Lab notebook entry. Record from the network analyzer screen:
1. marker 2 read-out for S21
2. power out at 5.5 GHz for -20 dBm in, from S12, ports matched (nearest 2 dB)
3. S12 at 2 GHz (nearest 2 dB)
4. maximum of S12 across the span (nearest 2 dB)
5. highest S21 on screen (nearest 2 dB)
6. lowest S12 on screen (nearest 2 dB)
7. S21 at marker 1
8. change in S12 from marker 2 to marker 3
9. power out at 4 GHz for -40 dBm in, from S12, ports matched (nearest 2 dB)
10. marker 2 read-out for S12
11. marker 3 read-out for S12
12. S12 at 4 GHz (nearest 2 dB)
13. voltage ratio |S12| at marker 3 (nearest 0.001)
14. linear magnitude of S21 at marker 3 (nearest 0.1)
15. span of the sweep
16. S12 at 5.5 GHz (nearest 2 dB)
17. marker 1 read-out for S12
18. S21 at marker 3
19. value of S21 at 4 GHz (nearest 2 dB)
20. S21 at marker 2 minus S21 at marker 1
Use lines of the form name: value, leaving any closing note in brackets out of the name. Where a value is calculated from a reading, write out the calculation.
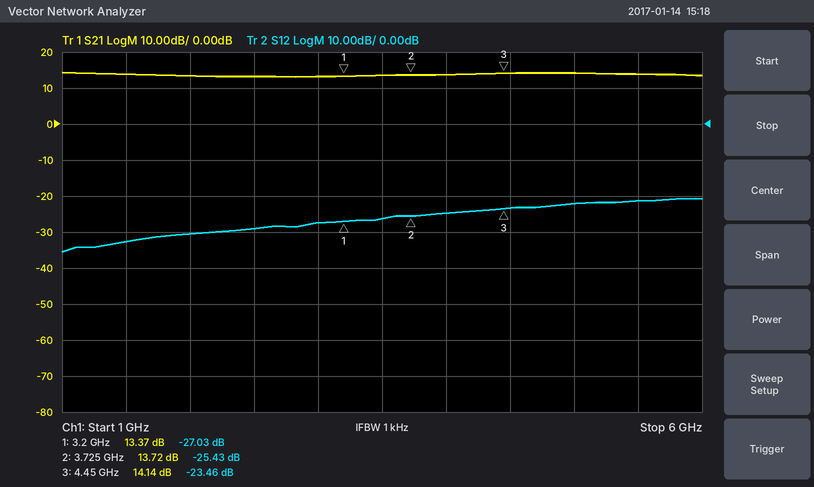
marker 2 read-out for S21: 13.72 dB
power out at 5.5 GHz for -20 dBm in, from S12, ports matched: -20 dBm + (-22 dB) = -42 dBm
S12 at 2 GHz: -30 dB
maximum of S12 across the span: -20 dB
highest S21 on screen: 14 dB
lowest S12 on screen: -36 dB
S21 at marker 1: 13.37 dB
change in S12 from marker 2 to marker 3: -23.46 − (-25.43) = 1.97 dB
power out at 4 GHz for -40 dBm in, from S12, ports matched: -40 dBm + (-24 dB) = -64 dBm
marker 2 read-out for S12: -25.43 dB
marker 3 read-out for S12: -23.46 dB
S12 at 4 GHz: -24 dB
voltage ratio |S12| at marker 3: 10^(-23.46/20) ≈ 0.067
linear magnitude of S21 at marker 3: 10^(14.14/20) ≈ 5.1
span of the sweep: 5 GHz
S12 at 5.5 GHz: -22 dB
marker 1 read-out for S12: -27.03 dB
S21 at marker 3: 14.14 dB
value of S21 at 4 GHz: 14 dB
S21 at marker 2 minus S21 at marker 1: 13.72 − (13.37) = 0.35 dB
